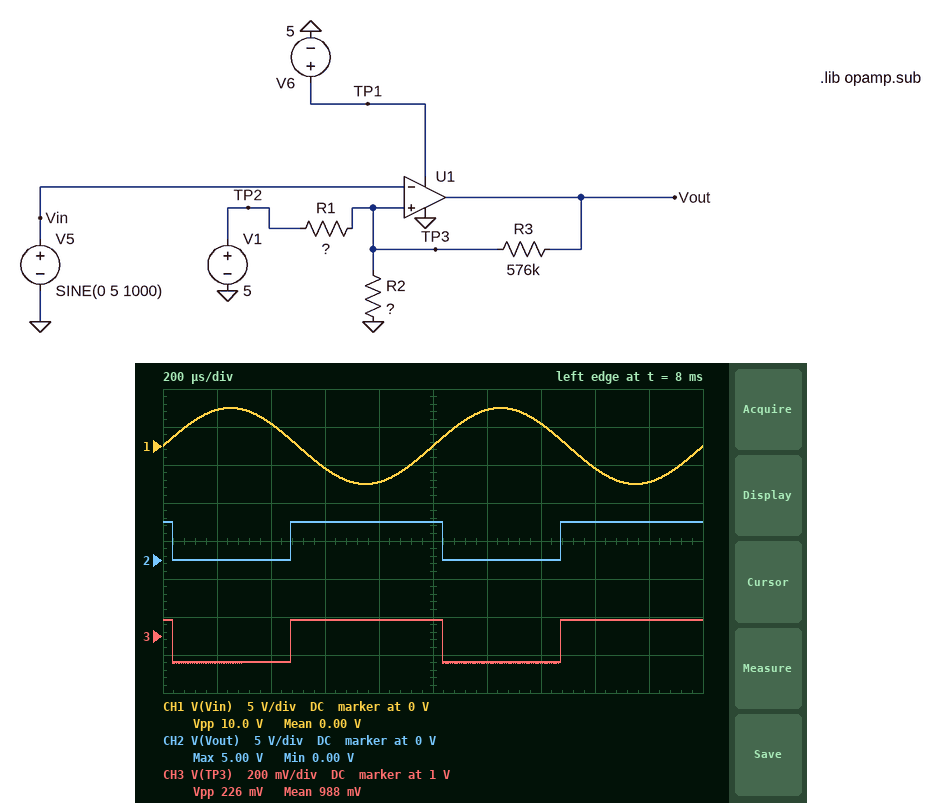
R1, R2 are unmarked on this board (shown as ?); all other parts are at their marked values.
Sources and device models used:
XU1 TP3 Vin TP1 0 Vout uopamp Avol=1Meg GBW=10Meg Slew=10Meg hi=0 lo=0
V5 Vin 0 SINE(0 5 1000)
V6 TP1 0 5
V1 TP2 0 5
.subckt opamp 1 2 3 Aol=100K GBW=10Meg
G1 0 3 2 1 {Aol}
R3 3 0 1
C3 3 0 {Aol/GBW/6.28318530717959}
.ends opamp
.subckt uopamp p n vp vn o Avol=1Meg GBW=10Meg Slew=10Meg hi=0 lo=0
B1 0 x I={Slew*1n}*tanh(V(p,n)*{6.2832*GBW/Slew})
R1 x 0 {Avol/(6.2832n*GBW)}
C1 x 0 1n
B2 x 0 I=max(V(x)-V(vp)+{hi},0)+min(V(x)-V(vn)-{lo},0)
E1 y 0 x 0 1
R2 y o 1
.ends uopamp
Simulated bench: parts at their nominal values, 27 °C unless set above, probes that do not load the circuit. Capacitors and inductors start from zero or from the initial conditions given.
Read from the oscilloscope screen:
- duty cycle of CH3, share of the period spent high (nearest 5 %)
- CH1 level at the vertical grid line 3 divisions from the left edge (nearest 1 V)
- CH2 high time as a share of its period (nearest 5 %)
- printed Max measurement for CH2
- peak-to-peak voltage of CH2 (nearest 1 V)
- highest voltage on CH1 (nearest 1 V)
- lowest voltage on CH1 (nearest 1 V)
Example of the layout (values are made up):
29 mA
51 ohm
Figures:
55 %
-3 V
55 %
5.00 V
5 V
5 V
-5 V
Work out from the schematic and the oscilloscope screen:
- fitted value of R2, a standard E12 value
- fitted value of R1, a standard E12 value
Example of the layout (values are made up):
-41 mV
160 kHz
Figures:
33 kΩ
150 kΩ
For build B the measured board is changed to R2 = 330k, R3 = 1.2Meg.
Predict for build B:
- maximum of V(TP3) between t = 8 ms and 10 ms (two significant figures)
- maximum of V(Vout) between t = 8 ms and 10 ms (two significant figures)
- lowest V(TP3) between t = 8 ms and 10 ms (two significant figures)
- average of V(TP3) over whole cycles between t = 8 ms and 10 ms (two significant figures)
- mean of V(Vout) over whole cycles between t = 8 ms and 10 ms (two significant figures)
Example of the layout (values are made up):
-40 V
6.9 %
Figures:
3.6 V
5.0 V
3.2 V
3.5 V
3.7 V
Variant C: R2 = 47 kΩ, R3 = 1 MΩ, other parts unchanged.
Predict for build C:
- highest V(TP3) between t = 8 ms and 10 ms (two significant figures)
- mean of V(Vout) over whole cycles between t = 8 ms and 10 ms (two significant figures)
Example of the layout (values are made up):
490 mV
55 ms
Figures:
1.3 V
2.9 V
